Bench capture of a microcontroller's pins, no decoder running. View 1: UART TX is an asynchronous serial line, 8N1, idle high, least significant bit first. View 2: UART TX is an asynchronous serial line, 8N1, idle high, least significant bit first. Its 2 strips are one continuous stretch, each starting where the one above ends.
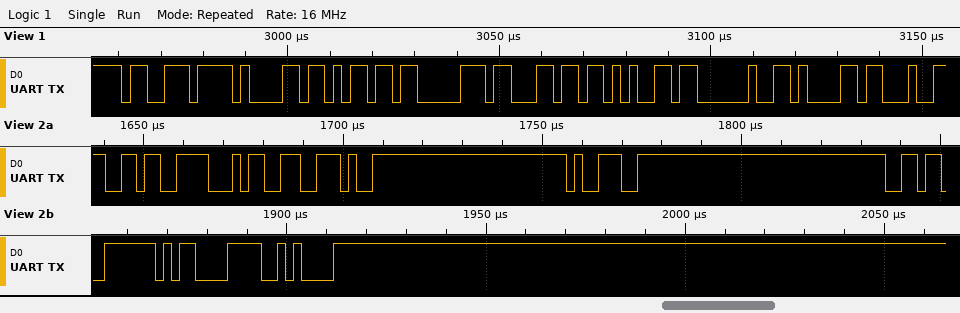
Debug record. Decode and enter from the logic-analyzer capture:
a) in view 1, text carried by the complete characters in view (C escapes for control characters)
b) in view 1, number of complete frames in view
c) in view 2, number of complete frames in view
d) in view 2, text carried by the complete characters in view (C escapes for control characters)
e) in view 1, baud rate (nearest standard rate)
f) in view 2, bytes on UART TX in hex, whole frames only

"sample a"
8
7
"64.96\r\n"
500000 baud
0x36 0x34 0x2E 0x39 0x36 0x0D 0x0A
